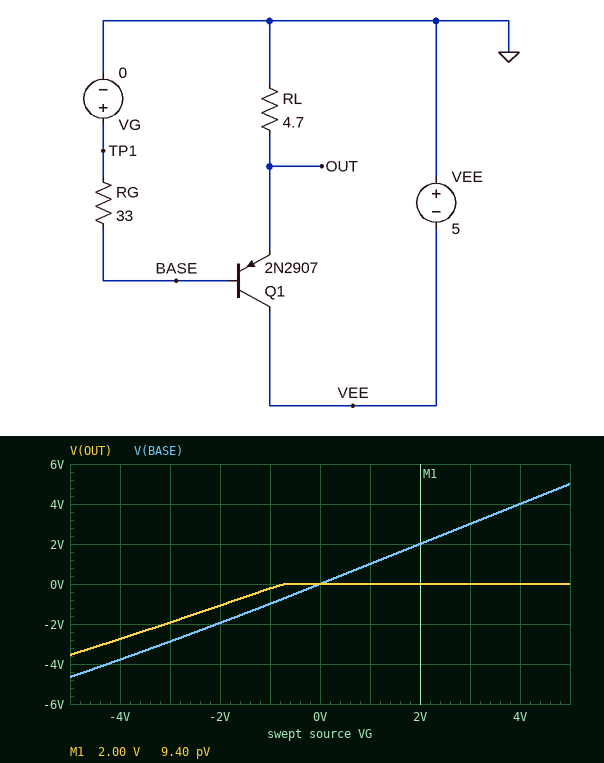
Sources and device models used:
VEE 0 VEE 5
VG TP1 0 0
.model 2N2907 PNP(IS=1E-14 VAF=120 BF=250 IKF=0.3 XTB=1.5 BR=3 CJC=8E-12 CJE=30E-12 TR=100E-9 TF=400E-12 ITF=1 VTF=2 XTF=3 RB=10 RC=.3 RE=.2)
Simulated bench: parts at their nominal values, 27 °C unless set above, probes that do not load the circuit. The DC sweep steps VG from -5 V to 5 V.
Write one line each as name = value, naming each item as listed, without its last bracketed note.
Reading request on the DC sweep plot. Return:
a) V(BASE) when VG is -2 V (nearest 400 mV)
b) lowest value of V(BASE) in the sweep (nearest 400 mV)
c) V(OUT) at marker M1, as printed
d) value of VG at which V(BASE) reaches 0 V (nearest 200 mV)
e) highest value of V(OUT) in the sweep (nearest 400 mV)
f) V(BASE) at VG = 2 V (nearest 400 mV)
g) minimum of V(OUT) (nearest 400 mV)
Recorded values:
V(BASE) when VG is -2 V = -2.0 V
lowest value of V(BASE) in the sweep = -4.8 V
V(OUT) at marker M1, as printed = 9.40 pV
value of VG at which V(BASE) reaches 0 V = 0 V
highest value of V(OUT) in the sweep = 0 V
V(BASE) at VG = 2 V = 2.0 V
minimum of V(OUT) = -3.6 V
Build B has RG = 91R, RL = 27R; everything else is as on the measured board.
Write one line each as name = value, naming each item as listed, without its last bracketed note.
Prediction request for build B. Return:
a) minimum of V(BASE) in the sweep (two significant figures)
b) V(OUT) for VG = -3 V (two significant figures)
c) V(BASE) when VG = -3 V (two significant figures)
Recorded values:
minimum of V(BASE) in the sweep = -4.9 V
V(OUT) for VG = -3 V = -2.2 V
V(BASE) when VG = -3 V = -3.0 V
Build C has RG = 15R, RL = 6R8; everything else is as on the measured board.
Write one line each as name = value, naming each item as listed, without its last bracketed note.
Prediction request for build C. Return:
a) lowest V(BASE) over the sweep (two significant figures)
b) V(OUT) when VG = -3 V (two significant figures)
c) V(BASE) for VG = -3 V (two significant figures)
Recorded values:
lowest V(BASE) over the sweep = -4.9 V
V(OUT) when VG = -3 V = -2.1 V
V(BASE) for VG = -3 V = -3.0 V
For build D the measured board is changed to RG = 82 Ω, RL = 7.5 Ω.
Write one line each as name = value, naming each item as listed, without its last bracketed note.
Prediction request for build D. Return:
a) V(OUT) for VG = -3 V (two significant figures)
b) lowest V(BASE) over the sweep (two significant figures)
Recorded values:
V(OUT) for VG = -3 V = -2.0 V
lowest V(BASE) over the sweep = -4.6 V
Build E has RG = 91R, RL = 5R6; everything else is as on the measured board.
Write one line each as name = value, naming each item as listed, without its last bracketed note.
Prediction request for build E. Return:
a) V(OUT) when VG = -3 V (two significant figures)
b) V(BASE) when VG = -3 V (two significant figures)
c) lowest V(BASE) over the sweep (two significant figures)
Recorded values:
V(OUT) when VG = -3 V = -1.8 V
V(BASE) when VG = -3 V = -2.8 V
lowest V(BASE) over the sweep = -4.4 V
